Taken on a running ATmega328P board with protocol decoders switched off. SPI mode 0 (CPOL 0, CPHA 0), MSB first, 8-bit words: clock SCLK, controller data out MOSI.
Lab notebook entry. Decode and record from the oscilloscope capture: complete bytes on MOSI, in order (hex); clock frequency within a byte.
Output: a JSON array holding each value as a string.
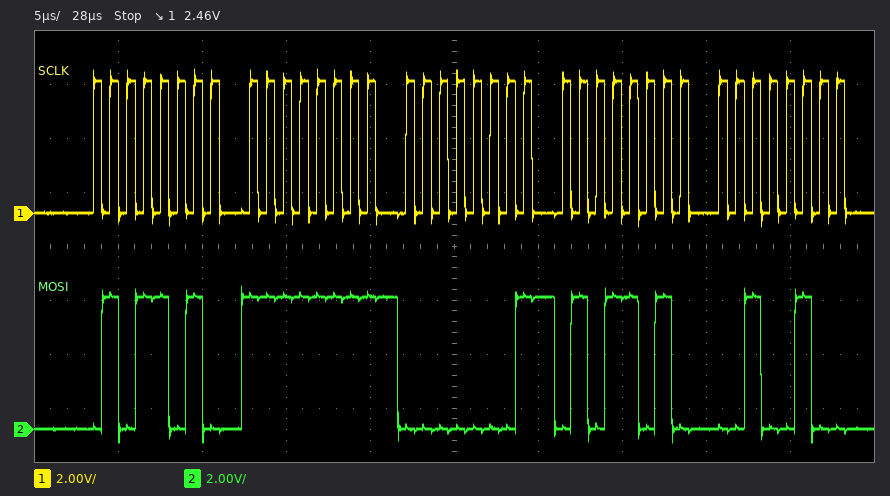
["0x5A 0xFF 0x01 0x5A 0x24", "1 MHz"]
